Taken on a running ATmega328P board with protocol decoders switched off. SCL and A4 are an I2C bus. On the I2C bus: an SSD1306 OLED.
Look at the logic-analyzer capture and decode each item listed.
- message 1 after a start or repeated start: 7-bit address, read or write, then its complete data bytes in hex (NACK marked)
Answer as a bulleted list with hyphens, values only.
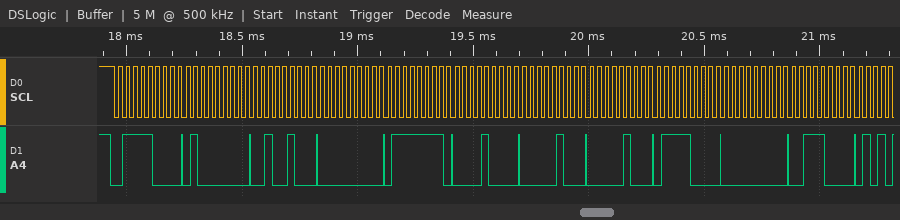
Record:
- 0x3C write: 40 24 00 7F 08 04 04 78 00 38
